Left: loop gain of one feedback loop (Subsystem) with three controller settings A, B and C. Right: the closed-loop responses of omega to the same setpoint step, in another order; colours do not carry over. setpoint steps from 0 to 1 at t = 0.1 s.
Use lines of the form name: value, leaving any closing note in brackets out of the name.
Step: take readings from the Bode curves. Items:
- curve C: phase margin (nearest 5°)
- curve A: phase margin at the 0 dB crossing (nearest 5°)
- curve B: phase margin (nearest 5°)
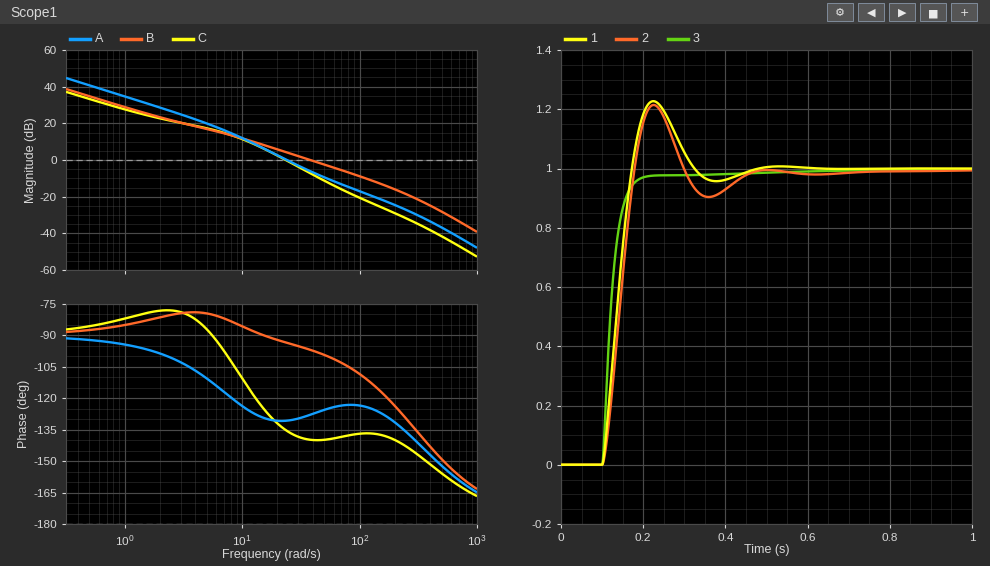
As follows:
curve C: phase margin: 45°
curve A: phase margin at the 0 dB crossing: 50°
curve B: phase margin: 85°
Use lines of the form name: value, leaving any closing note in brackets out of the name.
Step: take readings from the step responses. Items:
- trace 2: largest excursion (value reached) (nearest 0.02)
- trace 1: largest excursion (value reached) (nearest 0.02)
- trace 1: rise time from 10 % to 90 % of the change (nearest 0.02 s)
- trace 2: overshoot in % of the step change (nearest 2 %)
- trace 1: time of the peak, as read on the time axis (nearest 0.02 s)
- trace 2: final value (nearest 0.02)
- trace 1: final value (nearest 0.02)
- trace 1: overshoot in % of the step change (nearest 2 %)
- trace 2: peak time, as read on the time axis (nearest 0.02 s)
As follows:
trace 2: largest excursion (value reached): 1.22
trace 1: largest excursion (value reached): 1.22
trace 1: rise time from 10 % to 90 % of the change: 0.06 s
trace 2: overshoot in % of the step change: 22 %
trace 1: time of the peak, as read on the time axis: 0.22 s
trace 2: final value: 1.00
trace 1: final value: 1.00
trace 1: overshoot in % of the step change: 22 %
trace 2: peak time, as read on the time axis: 0.22 s
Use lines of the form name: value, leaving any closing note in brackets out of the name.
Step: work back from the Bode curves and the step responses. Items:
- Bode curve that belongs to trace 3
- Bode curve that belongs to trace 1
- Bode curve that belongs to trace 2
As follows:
Bode curve that belongs to trace 3: B
Bode curve that belongs to trace 1: A
Bode curve that belongs to trace 2: C
